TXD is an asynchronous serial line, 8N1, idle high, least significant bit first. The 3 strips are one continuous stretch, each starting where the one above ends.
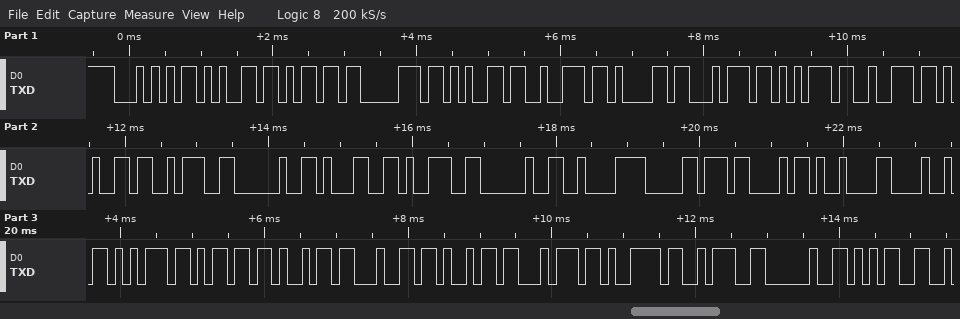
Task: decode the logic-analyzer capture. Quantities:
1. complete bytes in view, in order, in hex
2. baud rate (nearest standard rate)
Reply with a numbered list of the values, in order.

1. 54 65 6D 70 65 72 61 74 75 72 65 3A 20 31 39 20 C2 B0 43 09 48 75 6D 69 64 69 74 79 3A 20 35
2. 9600 baud
